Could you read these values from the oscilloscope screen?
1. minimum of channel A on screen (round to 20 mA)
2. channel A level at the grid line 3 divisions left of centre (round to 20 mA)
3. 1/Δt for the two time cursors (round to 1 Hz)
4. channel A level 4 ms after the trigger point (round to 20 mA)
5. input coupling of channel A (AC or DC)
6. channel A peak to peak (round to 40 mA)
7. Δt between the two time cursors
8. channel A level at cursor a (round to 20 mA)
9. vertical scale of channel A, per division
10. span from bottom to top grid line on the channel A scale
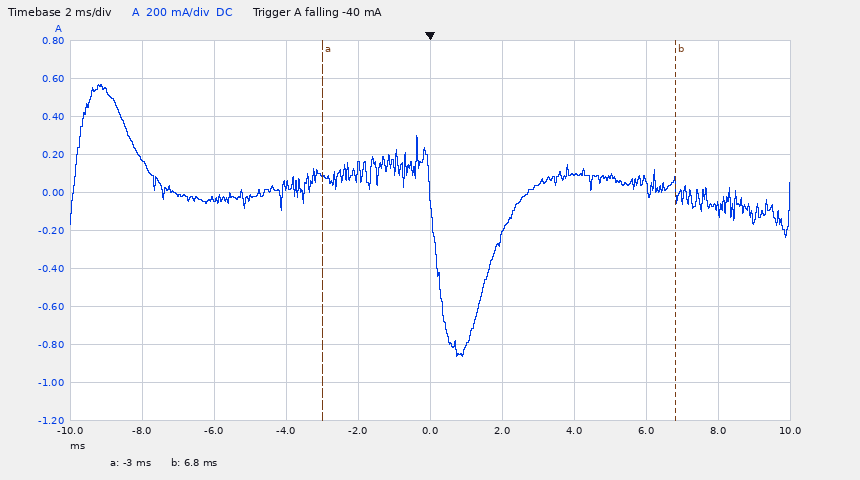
-860 mA
-40 mA
102 Hz
100 mA
DC
1.44 A
9.8 ms
80 mA
200 mA
2 A
